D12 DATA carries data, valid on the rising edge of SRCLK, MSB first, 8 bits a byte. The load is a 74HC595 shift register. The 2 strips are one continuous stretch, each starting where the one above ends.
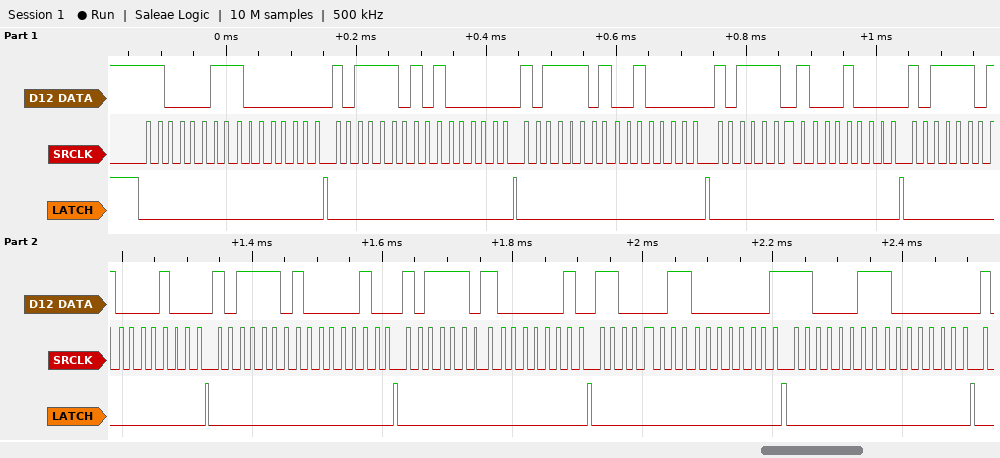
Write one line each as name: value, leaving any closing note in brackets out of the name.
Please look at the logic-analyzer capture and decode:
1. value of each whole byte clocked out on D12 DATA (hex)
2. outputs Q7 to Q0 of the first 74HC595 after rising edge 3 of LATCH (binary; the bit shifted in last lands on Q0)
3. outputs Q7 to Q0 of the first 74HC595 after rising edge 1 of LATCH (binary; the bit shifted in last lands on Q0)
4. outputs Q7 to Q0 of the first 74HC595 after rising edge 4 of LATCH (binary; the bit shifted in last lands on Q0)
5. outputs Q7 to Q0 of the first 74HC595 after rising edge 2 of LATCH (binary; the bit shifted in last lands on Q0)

value of each whole byte clocked out on D12 DATA: 0xC3 0x80 0xBD 0x40 0xBD 0x20 0xBD 0x10 0xBD 0x08 0xBD 0x04 0xBD 0x02 0xC3 0x01 0xC3 0x80
outputs Q7 to Q0 of the first 74HC595 after rising edge 3 of LATCH: 00100000
outputs Q7 to Q0 of the first 74HC595 after rising edge 1 of LATCH: 10000000
outputs Q7 to Q0 of the first 74HC595 after rising edge 4 of LATCH: 00010000
outputs Q7 to Q0 of the first 74HC595 after rising edge 2 of LATCH: 01000000
